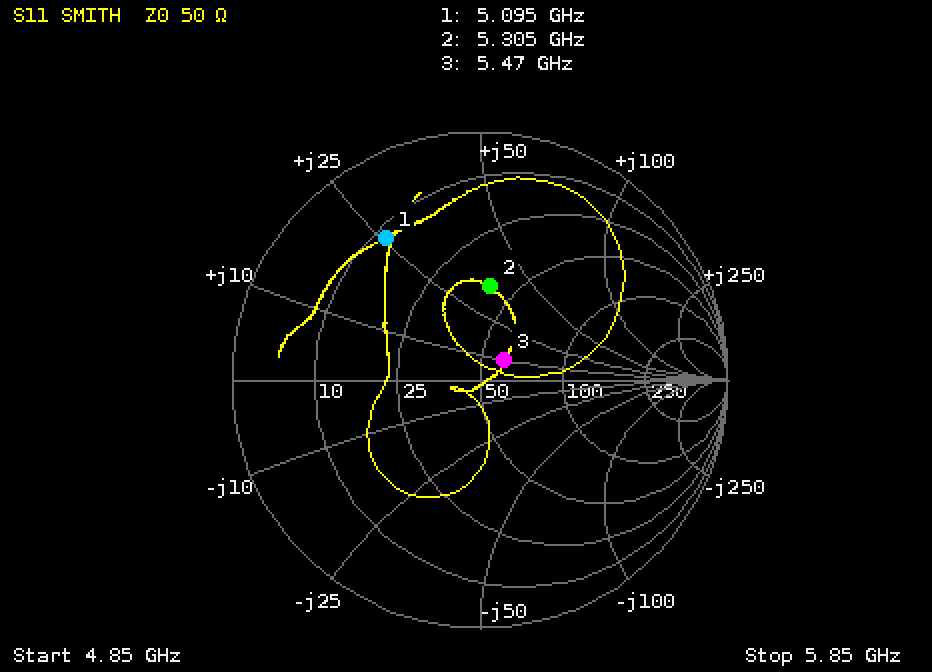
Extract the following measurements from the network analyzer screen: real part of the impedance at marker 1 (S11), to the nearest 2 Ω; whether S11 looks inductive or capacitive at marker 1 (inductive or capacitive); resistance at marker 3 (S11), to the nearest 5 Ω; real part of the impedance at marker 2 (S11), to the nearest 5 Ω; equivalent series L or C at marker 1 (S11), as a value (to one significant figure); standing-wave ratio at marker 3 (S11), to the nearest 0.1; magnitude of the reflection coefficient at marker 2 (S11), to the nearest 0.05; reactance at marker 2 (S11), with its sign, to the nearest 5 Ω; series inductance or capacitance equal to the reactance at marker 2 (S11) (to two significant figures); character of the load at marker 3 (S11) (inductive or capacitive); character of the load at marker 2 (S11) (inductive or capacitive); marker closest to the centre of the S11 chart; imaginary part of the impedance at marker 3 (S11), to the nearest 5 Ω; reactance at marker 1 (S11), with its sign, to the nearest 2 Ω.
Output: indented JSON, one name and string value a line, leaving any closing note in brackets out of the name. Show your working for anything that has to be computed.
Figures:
{
  "real part of the impedance at marker 1 (S11), to the nearest 2 Ω": "12 Ω",
  "whether S11 looks inductive or capacitive at marker 1": "inductive",
  "resistance at marker 3 (S11), to the nearest 5 Ω": "60 Ω",
  "real part of the impedance at marker 2 (S11), to the nearest 5 Ω": "40 Ω",
  "equivalent series L or C at marker 1 (S11), as a value": "L = 26 Ω/(2π × 5.095 GHz) ≈ 812 pH, so 800 pH to one significant figure",
  "standing-wave ratio at marker 3 (S11), to the nearest 0.1": "1.3",
  "magnitude of the reflection coefficient at marker 2 (S11), to the nearest 0.05": "0.40",
  "reactance at marker 2 (S11), with its sign, to the nearest 5 Ω": "+35 Ω",
  "series inductance or capacitance equal to the reactance at marker 2 (S11)": "L = 35 Ω/(2π × 5.305 GHz) ≈ 1.1 nH",
  "character of the load at marker 3 (S11)": "inductive",
  "character of the load at marker 2 (S11)": "inductive",
  "marker closest to the centre of the S11 chart": "marker 3",
  "imaginary part of the impedance at marker 3 (S11), to the nearest 5 Ω": "+10 Ω",
  "reactance at marker 1 (S11), with its sign, to the nearest 2 Ω": "+26 Ω"
}
